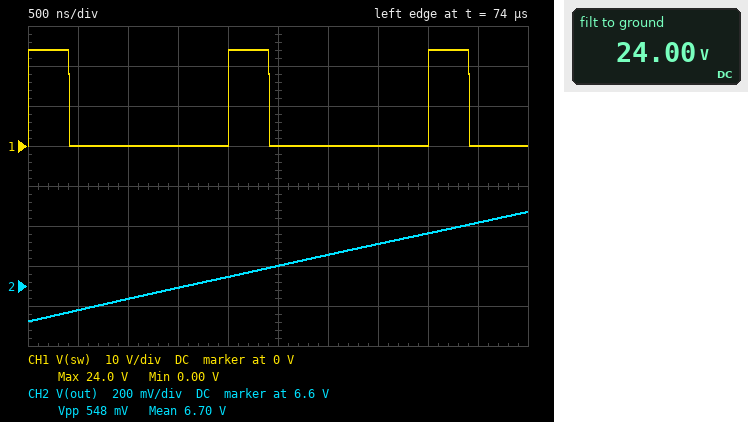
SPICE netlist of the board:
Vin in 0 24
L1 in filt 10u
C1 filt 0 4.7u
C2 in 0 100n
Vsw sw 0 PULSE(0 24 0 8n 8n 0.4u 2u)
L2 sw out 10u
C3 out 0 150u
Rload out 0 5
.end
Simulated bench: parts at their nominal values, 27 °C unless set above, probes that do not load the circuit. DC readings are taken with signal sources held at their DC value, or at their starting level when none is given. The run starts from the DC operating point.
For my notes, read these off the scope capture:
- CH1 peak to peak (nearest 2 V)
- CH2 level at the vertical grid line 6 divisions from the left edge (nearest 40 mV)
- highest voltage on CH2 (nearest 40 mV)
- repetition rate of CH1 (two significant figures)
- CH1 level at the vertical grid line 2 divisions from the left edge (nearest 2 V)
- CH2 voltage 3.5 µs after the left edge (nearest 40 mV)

24 V
6.76 V
6.96 V
500 kHz
0 V
6.80 V
